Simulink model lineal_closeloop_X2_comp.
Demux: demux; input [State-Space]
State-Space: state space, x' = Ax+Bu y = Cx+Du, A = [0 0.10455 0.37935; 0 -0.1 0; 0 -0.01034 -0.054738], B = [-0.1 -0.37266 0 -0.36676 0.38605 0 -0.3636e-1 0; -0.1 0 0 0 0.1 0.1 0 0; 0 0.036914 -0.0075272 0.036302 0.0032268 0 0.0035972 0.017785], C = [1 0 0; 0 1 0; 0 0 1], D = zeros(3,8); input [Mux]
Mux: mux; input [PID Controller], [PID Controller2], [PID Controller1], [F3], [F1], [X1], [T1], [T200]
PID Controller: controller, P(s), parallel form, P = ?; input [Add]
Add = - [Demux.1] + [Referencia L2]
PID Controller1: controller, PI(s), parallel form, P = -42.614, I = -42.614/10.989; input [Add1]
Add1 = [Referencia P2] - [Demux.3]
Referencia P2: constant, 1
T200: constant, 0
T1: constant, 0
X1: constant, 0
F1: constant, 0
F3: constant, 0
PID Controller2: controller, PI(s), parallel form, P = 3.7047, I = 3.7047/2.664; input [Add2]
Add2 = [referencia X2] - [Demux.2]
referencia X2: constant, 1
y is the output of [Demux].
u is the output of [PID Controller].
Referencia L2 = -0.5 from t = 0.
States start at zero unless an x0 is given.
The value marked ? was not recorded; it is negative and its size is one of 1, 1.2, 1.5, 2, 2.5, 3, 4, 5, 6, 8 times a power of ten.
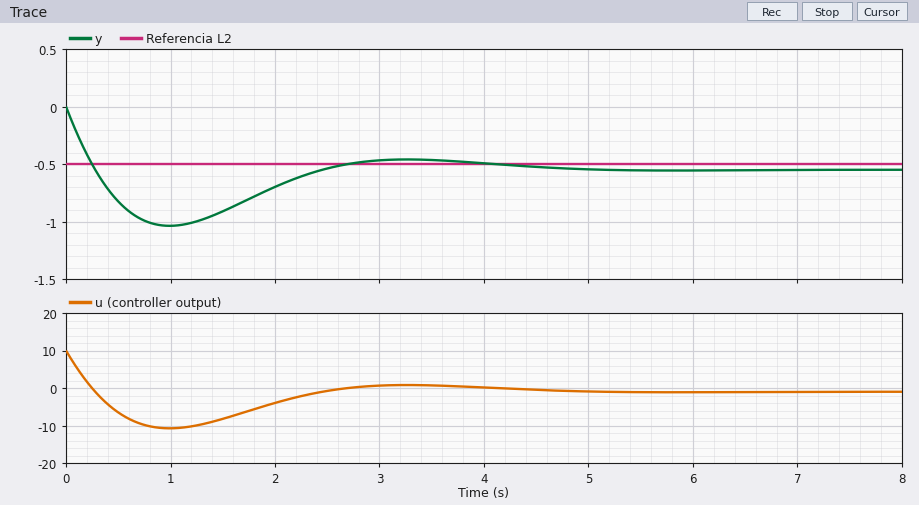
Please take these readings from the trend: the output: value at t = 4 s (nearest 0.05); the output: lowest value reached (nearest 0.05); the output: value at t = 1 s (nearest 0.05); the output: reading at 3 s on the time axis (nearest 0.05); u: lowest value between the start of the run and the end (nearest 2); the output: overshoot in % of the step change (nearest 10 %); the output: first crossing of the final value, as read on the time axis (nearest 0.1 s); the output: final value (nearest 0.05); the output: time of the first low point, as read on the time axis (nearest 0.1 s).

-0.50
-1.05
-1.05
-0.45
-10
90 %
0.3 s
-0.55
1.0 s
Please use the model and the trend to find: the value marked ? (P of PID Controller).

-20
